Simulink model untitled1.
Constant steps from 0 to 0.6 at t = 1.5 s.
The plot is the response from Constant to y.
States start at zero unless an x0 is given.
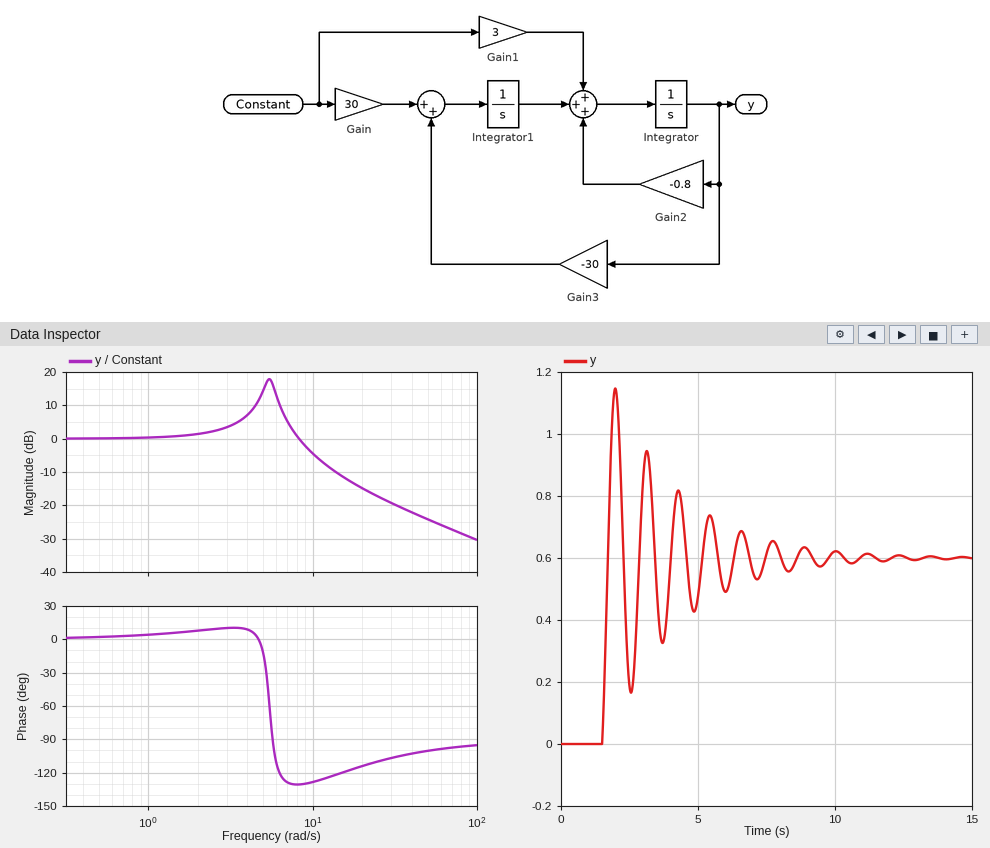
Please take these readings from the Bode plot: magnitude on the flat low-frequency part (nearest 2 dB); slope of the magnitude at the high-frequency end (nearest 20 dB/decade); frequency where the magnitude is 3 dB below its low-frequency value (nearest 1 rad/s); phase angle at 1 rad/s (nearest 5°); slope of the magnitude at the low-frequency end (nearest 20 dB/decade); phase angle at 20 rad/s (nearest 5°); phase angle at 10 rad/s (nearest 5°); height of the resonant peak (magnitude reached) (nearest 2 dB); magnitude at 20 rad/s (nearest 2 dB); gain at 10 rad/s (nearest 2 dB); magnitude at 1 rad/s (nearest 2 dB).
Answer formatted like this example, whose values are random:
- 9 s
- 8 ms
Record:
- 0 dB
- -20 dB/decade
- 9 rad/s
- 5°
- 0 dB/decade
- -115°
- -130°
- 18 dB
- -14 dB
- -4 dB
- 0 dB
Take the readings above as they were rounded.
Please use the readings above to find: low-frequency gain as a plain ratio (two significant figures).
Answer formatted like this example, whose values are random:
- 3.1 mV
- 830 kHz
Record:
- 1.0
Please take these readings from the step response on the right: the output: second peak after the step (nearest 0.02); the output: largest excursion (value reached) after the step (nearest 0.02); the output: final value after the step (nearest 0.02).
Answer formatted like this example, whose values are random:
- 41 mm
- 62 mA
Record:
- 0.94
- 1.14
- 0.60
